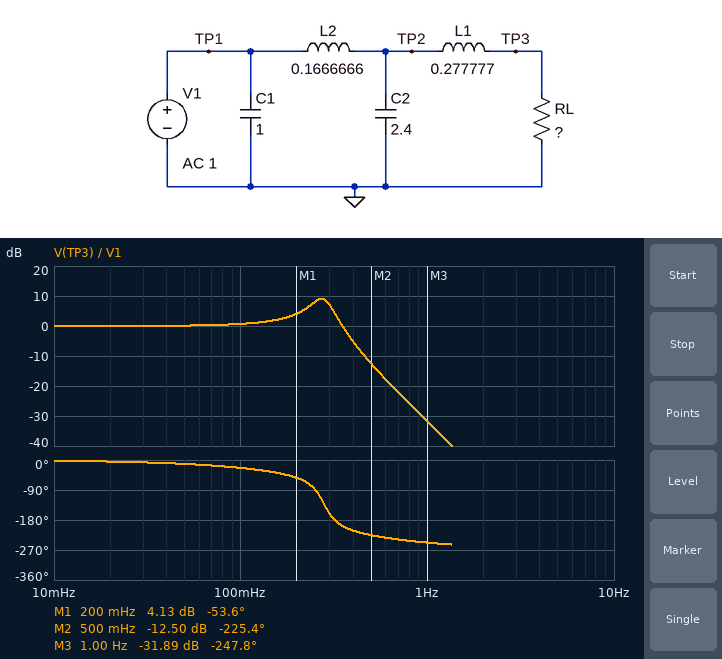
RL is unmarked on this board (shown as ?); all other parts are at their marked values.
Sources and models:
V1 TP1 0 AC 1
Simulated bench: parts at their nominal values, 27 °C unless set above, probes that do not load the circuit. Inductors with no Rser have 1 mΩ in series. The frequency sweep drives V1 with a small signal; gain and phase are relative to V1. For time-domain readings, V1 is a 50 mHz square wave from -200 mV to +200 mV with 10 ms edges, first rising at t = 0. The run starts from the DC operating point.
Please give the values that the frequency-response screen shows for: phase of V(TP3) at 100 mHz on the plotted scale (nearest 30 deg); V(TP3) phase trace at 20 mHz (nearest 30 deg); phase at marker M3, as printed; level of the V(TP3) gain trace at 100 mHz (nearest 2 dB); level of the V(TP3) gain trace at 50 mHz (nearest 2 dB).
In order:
-30 deg
0 deg
-247.8 deg
0 dB
0 dB
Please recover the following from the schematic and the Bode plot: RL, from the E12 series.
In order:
0.68 Ω
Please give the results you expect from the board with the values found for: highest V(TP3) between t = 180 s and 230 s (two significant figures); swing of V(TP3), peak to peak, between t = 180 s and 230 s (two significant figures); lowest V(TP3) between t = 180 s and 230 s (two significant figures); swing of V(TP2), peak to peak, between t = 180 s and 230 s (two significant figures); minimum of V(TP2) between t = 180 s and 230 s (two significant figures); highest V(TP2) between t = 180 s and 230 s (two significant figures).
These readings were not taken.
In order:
390 mV
770 mV
-390 mV
870 mV
-440 mV
440 mV
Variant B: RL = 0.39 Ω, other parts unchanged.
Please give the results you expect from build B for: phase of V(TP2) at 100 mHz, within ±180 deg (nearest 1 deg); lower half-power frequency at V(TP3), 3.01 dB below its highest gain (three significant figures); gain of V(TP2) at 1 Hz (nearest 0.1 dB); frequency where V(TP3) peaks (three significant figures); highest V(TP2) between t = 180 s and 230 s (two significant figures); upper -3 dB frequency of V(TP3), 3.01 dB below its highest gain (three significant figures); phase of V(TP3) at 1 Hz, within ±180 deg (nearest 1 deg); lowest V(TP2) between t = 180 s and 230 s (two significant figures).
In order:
-13 deg
251 mHz
-23.1 dB
294 mHz
370 mV
325 mHz
103 deg
-370 mV
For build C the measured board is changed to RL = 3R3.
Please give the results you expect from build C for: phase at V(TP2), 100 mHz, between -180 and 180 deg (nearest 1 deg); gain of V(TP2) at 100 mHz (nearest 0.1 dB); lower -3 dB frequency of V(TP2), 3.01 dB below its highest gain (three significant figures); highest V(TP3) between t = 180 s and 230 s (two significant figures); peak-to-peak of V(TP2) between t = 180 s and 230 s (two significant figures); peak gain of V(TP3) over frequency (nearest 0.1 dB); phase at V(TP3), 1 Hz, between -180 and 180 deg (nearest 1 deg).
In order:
-2 deg
1.5 dB
242 mHz
910 mV
1.8 V
21.6 dB
153 deg
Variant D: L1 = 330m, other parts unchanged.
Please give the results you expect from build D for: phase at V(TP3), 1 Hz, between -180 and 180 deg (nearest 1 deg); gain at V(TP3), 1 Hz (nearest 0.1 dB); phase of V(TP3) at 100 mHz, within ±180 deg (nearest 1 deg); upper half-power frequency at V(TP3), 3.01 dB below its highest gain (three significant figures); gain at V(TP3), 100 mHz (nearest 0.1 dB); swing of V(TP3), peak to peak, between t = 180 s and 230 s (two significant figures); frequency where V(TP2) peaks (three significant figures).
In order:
109 deg
-33.3 dB
-26 deg
304 mHz
0.5 dB
750 mV
276 mHz
